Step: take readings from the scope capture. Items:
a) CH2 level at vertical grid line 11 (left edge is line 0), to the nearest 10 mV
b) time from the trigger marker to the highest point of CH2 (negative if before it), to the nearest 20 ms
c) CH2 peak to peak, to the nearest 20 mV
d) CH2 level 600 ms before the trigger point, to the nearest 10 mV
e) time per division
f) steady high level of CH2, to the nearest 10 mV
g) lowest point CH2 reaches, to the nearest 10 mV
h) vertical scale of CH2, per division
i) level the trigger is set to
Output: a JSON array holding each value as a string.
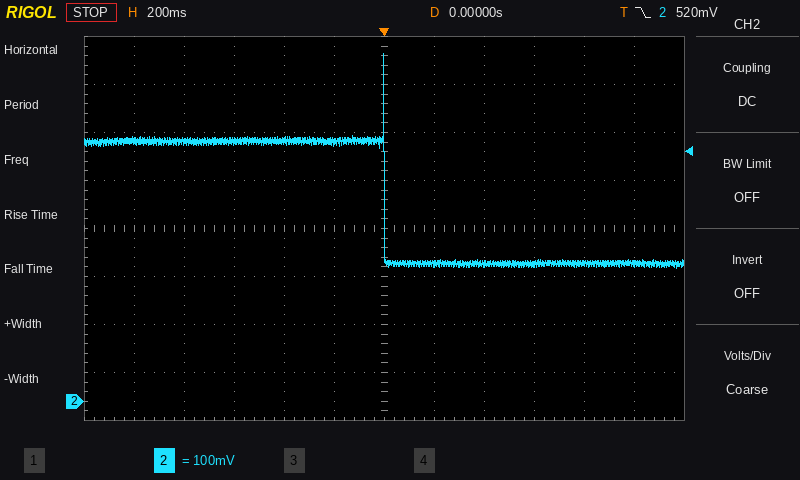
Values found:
["290 mV", "0 ms", "440 mV", "540 mV", "200 ms", "540 mV", "280 mV", "100 mV", "520 mV"]
